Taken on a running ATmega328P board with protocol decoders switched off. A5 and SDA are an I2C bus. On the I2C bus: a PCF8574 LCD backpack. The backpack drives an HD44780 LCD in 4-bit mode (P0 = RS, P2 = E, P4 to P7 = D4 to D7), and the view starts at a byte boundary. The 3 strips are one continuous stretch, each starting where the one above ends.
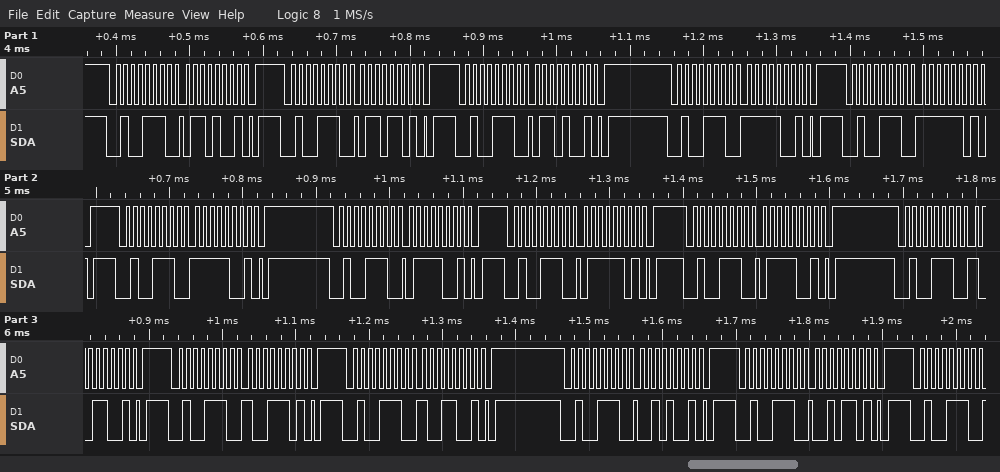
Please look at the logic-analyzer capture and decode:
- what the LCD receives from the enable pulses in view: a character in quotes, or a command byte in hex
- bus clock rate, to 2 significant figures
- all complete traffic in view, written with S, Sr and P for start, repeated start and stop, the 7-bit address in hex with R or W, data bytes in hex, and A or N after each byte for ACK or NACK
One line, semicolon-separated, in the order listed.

'o' 'y'; 100 kHz; S 27W A 69 A P S 27W A 6D A P S 27W A 69 A P S 27W A F9 A P S 27W A FD A P S 27W A F9 A P S 27W A 79 A P S 27W A 7D A P S 27W A 79 A P S 27W A 99 A P S 27W A 9D A P S 27W A 99 A P S 27W A 29 A P S 27W A 2D A P S 27W A
